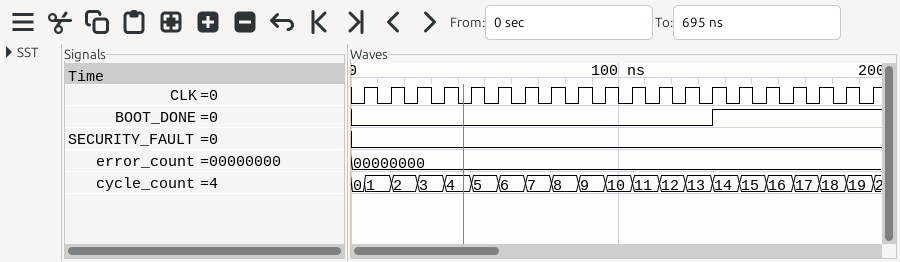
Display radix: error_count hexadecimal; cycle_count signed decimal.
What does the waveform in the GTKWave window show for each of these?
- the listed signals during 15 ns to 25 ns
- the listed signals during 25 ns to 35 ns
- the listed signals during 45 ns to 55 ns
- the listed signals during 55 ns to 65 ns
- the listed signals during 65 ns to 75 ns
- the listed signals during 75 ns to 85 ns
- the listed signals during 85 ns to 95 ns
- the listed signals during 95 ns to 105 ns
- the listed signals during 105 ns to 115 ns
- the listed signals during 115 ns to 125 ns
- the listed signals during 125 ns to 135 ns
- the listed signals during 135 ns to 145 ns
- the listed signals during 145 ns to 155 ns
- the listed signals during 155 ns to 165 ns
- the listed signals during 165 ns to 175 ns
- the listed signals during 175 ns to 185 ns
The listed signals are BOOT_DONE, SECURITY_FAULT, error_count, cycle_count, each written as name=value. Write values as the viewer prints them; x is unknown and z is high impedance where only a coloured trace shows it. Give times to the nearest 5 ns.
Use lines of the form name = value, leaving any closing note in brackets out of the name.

the listed signals during 15 ns to 25 ns = BOOT_DONE=0, SECURITY_FAULT=0, error_count=00000000, cycle_count=2
the listed signals during 25 ns to 35 ns = BOOT_DONE=0, SECURITY_FAULT=0, error_count=00000000, cycle_count=3
the listed signals during 45 ns to 55 ns = BOOT_DONE=0, SECURITY_FAULT=0, error_count=00000000, cycle_count=5
the listed signals during 55 ns to 65 ns = BOOT_DONE=0, SECURITY_FAULT=0, error_count=00000000, cycle_count=6
the listed signals during 65 ns to 75 ns = BOOT_DONE=0, SECURITY_FAULT=0, error_count=00000000, cycle_count=7
the listed signals during 75 ns to 85 ns = BOOT_DONE=0, SECURITY_FAULT=0, error_count=00000000, cycle_count=8
the listed signals during 85 ns to 95 ns = BOOT_DONE=0, SECURITY_FAULT=0, error_count=00000000, cycle_count=9
the listed signals during 95 ns to 105 ns = BOOT_DONE=0, SECURITY_FAULT=0, error_count=00000000, cycle_count=10
the listed signals during 105 ns to 115 ns = BOOT_DONE=0, SECURITY_FAULT=0, error_count=00000000, cycle_count=11
the listed signals during 115 ns to 125 ns = BOOT_DONE=0, SECURITY_FAULT=0, error_count=00000000, cycle_count=12
the listed signals during 125 ns to 135 ns = BOOT_DONE=0, SECURITY_FAULT=0, error_count=00000000, cycle_count=13
the listed signals during 135 ns to 145 ns = BOOT_DONE=1, SECURITY_FAULT=0, error_count=00000000, cycle_count=14
the listed signals during 145 ns to 155 ns = BOOT_DONE=1, SECURITY_FAULT=0, error_count=00000000, cycle_count=15
the listed signals during 155 ns to 165 ns = BOOT_DONE=1, SECURITY_FAULT=0, error_count=00000000, cycle_count=16
the listed signals during 165 ns to 175 ns = BOOT_DONE=1, SECURITY_FAULT=0, error_count=00000000, cycle_count=17
the listed signals during 175 ns to 185 ns = BOOT_DONE=1, SECURITY_FAULT=0, error_count=00000000, cycle_count=18
